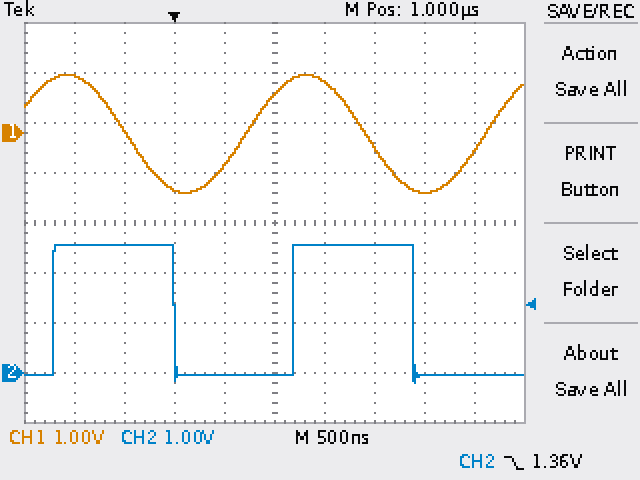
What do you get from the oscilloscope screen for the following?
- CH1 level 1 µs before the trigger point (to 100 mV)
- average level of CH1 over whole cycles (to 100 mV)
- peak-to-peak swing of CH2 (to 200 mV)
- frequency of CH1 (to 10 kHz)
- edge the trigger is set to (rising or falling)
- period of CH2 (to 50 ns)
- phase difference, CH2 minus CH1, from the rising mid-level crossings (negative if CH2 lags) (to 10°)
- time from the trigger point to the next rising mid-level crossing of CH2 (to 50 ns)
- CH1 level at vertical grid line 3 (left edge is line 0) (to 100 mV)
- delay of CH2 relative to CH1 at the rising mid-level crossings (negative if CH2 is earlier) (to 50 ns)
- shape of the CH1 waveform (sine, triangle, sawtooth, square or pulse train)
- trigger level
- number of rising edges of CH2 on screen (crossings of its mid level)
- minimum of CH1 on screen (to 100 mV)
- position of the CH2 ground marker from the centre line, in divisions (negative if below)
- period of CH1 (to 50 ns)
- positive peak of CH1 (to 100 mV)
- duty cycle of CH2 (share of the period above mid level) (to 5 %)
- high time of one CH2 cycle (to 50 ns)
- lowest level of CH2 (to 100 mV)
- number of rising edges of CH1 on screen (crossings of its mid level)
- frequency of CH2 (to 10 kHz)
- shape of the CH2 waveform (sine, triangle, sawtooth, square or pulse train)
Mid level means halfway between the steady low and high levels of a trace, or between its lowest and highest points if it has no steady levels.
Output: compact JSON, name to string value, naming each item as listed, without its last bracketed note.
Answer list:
{"CH1 level 1 µs before the trigger point": "1.1 V", "average level of CH1 over whole cycles": "0.0 V", "peak-to-peak swing of CH2": "2.8 V", "frequency of CH1": "420 kHz", "edge the trigger is set to": "falling", "period of CH2": "2.40 µs", "phase difference, CH2 minus CH1, from the rising mid-level crossings (negative if CH2 lags)": "-70°", "time from the trigger point to the next rising mid-level crossing of CH2": "1.20 µs", "CH1 level at vertical grid line 3 (left edge is line 0)": "-1.1 V", "delay of CH2 relative to CH1 at the rising mid-level crossings (negative if CH2 is earlier)": "+450 ns", "shape of the CH1 waveform": "sine", "trigger level": "1.36 V", "number of rising edges of CH2 on screen": "2", "minimum of CH1 on screen": "-1.2 V", "position of the CH2 ground marker from the centre line, in divisions": "-3.0 div", "period of CH1": "2.40 µs", "positive peak of CH1": "1.2 V", "duty cycle of CH2 (share of the period above mid level)": "50 %", "high time of one CH2 cycle": "1.20 µs", "lowest level of CH2": "-200 mV", "number of rising edges of CH1 on screen": "2", "frequency of CH2": "420 kHz", "shape of the CH2 waveform": "square"}
